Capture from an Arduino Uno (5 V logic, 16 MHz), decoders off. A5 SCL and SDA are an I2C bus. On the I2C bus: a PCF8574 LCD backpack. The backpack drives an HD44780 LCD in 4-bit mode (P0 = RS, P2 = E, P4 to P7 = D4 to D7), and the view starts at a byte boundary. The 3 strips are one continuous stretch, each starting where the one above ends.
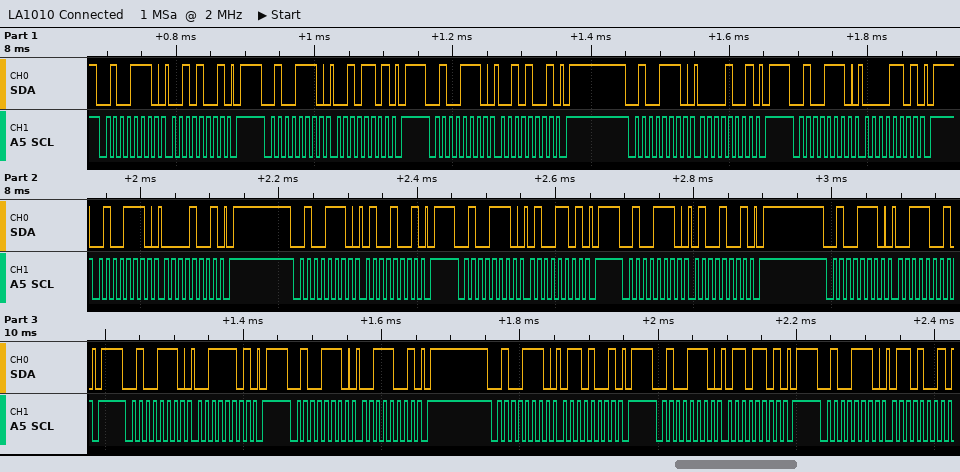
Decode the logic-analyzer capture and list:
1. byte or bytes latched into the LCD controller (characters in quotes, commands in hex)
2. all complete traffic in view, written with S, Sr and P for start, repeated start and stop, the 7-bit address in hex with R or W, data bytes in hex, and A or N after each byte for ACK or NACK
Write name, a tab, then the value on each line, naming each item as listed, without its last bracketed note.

byte or bytes latched into the LCD controller	' ' 'C'
all complete traffic in view, written with S, Sr and P for start, repeated start and stop, the 7-bit address in hex with R or W, data bytes in hex, and A or N after each byte for ACK or NACK	S 27W A 29 A P S 27W A 2D A P S 27W A 29 A P S 27W A 09 A P S 27W A 0D A P S 27W A 09 A P S 27W A 49 A P S 27W A 4D A P S 27W A 49 A P S 27W A 39 A P S 27W A 3D A P S 27W A 39 A P S 27W A 69 A P S 27W A 6D A P S 27W A 69 A
